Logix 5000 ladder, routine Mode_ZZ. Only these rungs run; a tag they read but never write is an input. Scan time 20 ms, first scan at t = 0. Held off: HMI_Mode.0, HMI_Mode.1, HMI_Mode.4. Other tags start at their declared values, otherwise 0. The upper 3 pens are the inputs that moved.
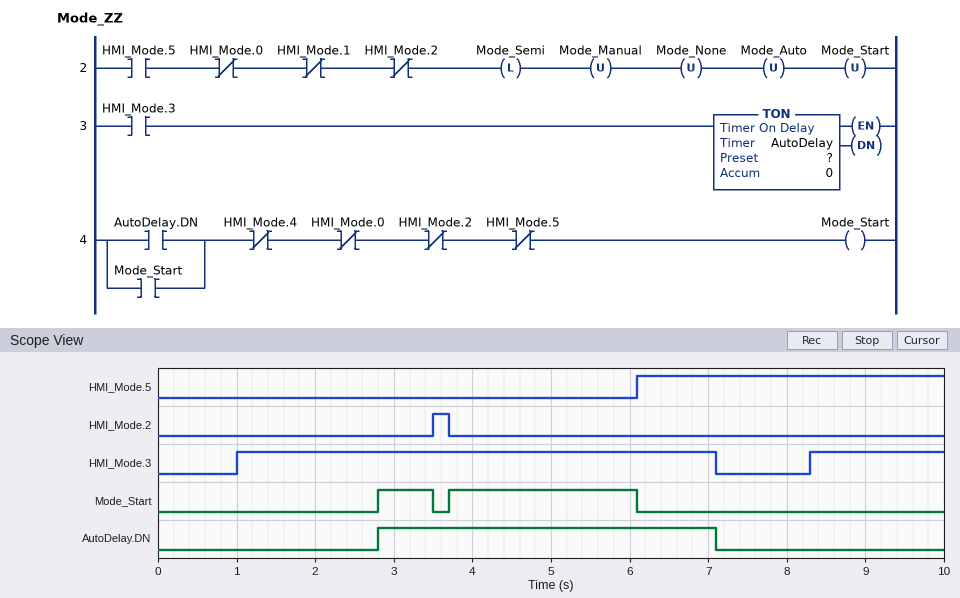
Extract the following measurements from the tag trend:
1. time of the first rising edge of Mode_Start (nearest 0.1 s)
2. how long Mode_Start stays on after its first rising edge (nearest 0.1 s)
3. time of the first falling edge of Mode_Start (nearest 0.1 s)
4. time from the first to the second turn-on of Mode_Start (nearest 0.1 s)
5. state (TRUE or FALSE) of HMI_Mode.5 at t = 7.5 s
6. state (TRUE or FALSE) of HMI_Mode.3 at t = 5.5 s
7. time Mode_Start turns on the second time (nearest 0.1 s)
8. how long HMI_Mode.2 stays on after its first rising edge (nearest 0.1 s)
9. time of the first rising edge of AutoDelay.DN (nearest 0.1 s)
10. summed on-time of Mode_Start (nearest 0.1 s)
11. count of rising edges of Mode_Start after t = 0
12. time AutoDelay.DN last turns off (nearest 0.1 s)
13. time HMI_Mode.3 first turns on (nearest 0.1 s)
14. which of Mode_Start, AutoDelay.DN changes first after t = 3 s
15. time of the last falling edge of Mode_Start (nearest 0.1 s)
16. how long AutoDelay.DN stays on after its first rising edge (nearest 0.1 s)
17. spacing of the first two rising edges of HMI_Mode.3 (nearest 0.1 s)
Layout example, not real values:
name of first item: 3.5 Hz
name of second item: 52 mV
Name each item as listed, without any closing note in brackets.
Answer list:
time of the first rising edge of Mode_Start: 2.8 s
how long Mode_Start stays on after its first rising edge: 0.7 s
time of the first falling edge of Mode_Start: 3.5 s
time from the first to the second turn-on of Mode_Start: 0.9 s
state (TRUE or FALSE) of HMI_Mode.5 at t = 7.5 s: TRUE
state (TRUE or FALSE) of HMI_Mode.3 at t = 5.5 s: TRUE
time Mode_Start turns on the second time: 3.7 s
how long HMI_Mode.2 stays on after its first rising edge: 0.2 s
time of the first rising edge of AutoDelay.DN: 2.8 s
summed on-time of Mode_Start: 3.1 s
count of rising edges of Mode_Start after t = 0: 2
time AutoDelay.DN last turns off: 7.1 s
time HMI_Mode.3 first turns on: 1.0 s
which of Mode_Start, AutoDelay.DN changes first after t = 3 s: Mode_Start
time of the last falling edge of Mode_Start: 6.1 s
how long AutoDelay.DN stays on after its first rising edge: 4.3 s
spacing of the first two rising edges of HMI_Mode.3: 7.3 s
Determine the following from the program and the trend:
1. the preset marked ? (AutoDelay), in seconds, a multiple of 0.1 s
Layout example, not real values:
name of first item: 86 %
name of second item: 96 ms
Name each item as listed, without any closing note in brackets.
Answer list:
the preset marked ? (AutoDelay), in seconds, a multiple of 0.1 s: 1.8 s
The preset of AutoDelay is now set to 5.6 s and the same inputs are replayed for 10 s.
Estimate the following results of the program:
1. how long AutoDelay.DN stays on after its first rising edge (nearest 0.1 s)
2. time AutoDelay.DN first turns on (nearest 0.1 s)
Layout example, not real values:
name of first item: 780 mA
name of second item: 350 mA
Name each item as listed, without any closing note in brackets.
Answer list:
how long AutoDelay.DN stays on after its first rising edge: 0.5 s
time AutoDelay.DN first turns on: 6.6 s
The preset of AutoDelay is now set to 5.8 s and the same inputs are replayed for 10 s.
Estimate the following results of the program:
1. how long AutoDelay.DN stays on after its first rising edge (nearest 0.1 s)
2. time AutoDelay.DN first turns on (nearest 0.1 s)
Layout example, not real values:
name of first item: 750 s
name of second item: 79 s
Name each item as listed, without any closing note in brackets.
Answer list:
how long AutoDelay.DN stays on after its first rising edge: 0.3 s
time AutoDelay.DN first turns on: 6.8 s
